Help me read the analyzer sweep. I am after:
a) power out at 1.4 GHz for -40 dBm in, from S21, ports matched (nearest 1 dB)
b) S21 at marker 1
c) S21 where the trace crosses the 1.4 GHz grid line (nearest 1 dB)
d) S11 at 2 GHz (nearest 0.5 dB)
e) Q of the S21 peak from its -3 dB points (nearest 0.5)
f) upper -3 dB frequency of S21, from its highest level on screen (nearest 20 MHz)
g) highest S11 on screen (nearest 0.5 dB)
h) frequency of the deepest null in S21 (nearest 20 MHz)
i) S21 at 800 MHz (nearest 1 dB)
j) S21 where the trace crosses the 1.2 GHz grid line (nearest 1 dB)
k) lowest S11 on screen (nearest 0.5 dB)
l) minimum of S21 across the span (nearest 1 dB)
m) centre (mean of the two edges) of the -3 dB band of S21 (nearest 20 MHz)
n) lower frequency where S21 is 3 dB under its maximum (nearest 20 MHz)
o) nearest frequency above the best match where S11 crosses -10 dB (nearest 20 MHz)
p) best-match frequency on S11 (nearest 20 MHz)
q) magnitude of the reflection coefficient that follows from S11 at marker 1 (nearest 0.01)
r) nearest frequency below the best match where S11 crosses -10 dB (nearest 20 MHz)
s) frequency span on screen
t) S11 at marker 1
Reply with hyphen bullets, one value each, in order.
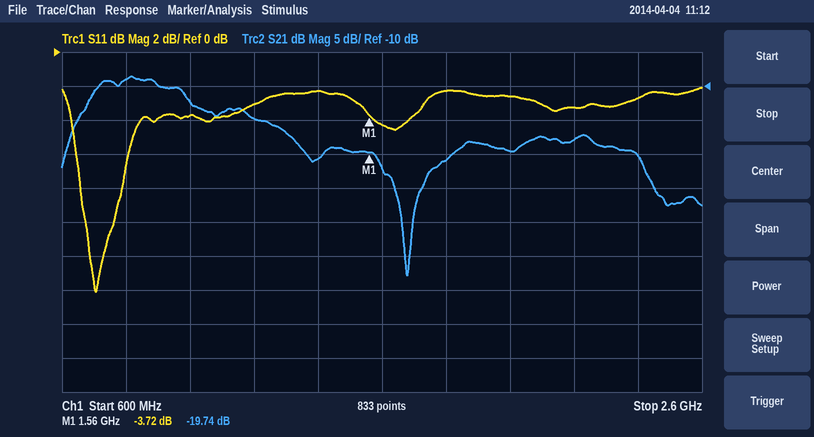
- -61 dBm
- -19.74 dB
- -21 dB
- -2.5 dB
- 3.0
- 980 MHz
- -2.0 dB
- 1.68 GHz
- -9 dB
- -15 dB
- -14.0 dB
- -38 dB
- 840 MHz
- 700 MHz
- 760 MHz
- 700 MHz
- 0.65
- 680 MHz
- 2 GHz
- -3.72 dB
